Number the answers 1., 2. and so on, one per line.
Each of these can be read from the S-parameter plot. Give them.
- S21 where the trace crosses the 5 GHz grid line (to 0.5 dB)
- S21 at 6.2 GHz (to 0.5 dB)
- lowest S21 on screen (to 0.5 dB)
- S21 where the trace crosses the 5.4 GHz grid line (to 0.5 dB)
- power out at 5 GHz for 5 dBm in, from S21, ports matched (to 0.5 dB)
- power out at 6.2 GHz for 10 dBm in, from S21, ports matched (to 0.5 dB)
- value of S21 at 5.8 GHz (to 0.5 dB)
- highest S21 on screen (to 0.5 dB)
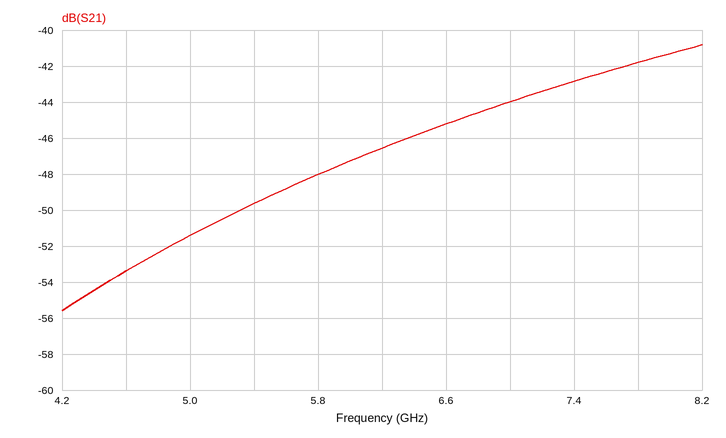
1. -51.5 dB
2. -46.5 dB
3. -55.5 dB
4. -49.5 dB
5. -46.5 dBm
6. -36.5 dBm
7. -48.0 dB
8. -41.0 dB
